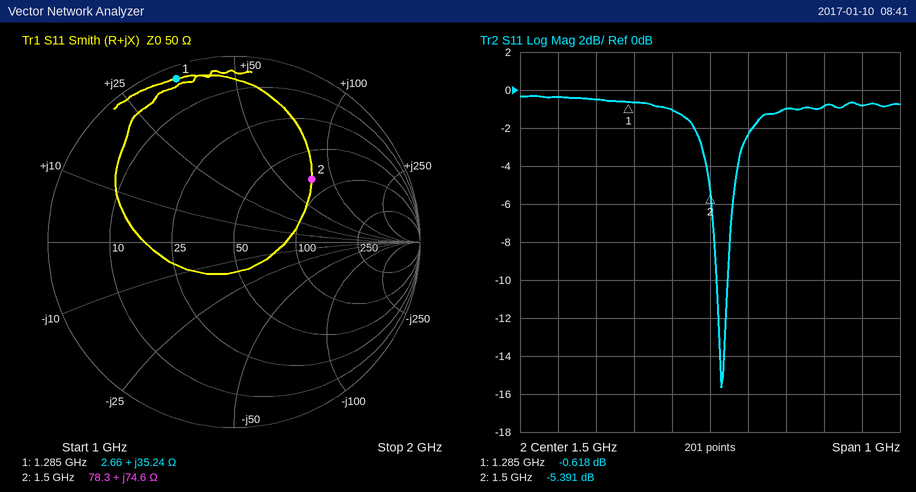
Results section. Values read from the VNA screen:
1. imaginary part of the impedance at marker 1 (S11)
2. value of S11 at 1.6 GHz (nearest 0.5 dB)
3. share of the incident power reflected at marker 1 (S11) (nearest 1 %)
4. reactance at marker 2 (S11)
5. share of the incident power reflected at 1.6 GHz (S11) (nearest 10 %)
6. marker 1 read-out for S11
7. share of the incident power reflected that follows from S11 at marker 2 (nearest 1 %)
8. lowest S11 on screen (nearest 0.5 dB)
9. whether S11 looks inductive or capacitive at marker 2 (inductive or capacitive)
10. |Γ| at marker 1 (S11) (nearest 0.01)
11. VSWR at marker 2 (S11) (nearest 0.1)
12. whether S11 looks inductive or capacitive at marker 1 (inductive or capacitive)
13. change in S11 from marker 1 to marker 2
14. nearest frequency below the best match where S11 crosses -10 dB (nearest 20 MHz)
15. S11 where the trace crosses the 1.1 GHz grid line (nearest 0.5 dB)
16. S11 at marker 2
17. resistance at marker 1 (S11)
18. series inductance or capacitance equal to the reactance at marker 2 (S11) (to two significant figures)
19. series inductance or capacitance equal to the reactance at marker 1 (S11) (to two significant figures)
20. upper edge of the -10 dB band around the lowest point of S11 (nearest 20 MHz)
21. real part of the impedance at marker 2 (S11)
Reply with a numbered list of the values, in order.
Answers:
1. +35.24 Ω
2. -2.5 dB
3. 87 %
4. +74.6 Ω
5. 60 %
6. -0.618 dB
7. 29 %
8. -15.5 dB
9. inductive
10. 0.93
11. 3.3
12. inductive
13. -4.773 dB
14. 1.52 GHz
15. -0.5 dB
16. -5.391 dB
17. 2.66 Ω
18. 7.9 nH
19. 4.4 nH
20. 1.54 GHz
21. 78.3 Ω
